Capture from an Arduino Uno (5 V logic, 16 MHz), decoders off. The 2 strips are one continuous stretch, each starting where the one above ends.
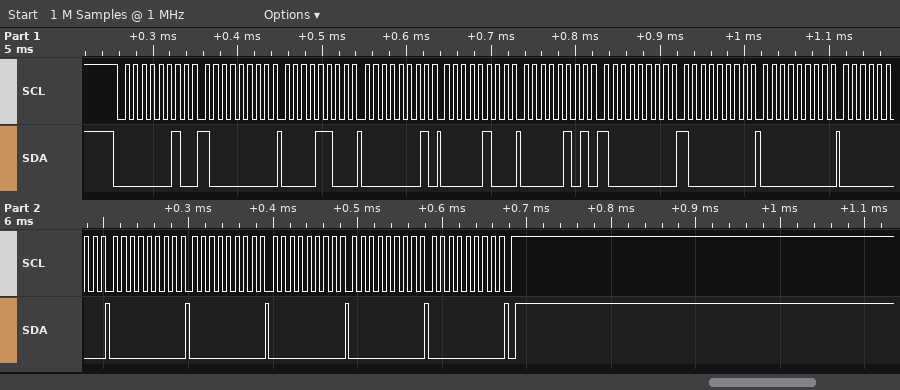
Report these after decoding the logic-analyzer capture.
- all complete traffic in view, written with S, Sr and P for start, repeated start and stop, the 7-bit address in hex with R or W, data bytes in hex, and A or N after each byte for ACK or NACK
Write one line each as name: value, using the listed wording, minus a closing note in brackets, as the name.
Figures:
all complete traffic in view, written with S, Sr and P for start, repeated start and stop, the 7-bit address in hex with R or W, data bytes in hex, and A or N after each byte for ACK or NACK: S 01W A 80 A 0C A 01 A 04 A 05 A 80 A 80 A 00 A 00 A 00 A 00 A 00 A 00 A 00 A P
